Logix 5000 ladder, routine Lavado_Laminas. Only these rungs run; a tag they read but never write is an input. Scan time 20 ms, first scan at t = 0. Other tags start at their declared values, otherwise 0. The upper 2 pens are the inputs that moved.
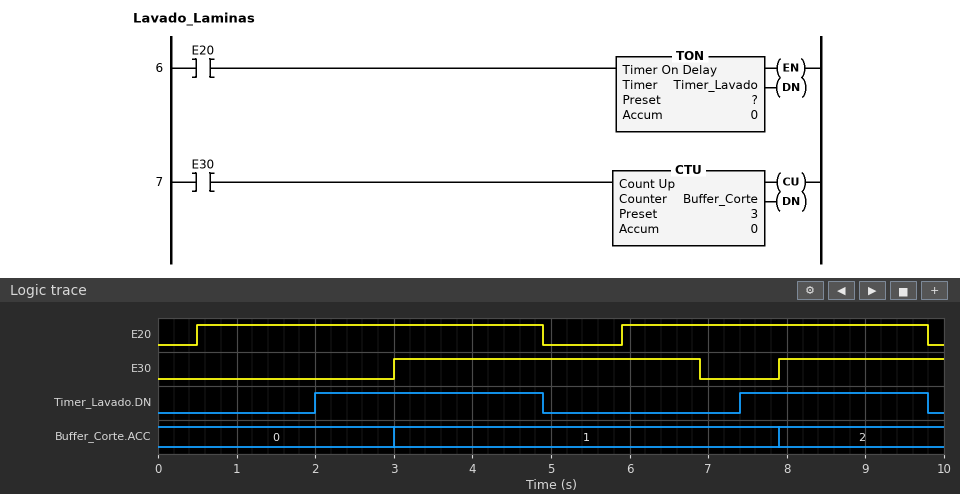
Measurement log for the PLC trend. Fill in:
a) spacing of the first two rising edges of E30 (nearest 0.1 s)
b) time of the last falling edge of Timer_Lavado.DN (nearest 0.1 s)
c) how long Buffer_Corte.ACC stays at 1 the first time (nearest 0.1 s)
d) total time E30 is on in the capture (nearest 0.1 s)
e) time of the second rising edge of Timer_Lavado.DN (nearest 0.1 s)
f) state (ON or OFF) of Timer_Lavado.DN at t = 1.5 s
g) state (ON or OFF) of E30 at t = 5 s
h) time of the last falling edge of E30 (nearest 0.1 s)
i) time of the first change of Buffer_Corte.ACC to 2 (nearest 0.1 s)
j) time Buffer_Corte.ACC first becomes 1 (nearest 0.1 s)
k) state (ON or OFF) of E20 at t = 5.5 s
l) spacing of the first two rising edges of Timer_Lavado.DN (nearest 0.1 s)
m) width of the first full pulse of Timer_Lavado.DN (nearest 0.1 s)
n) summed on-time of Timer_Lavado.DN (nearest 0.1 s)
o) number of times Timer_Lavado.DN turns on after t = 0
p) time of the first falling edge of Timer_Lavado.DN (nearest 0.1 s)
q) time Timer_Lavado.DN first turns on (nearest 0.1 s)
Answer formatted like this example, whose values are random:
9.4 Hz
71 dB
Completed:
4.9 s
9.8 s
4.9 s
6.0 s
7.4 s
OFF
ON
6.9 s
7.9 s
3.0 s
OFF
5.4 s
2.9 s
5.3 s
2
4.9 s
2.0 s
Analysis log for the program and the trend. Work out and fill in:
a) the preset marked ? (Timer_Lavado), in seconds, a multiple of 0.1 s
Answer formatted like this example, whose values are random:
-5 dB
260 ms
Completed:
1.5 s
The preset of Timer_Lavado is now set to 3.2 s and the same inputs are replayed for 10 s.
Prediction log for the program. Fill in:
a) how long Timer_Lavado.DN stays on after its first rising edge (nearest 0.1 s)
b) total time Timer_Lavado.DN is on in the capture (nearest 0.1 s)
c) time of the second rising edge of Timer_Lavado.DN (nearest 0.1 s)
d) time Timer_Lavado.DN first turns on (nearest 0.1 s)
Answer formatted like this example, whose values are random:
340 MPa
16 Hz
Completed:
1.2 s
1.9 s
9.1 s
3.7 s
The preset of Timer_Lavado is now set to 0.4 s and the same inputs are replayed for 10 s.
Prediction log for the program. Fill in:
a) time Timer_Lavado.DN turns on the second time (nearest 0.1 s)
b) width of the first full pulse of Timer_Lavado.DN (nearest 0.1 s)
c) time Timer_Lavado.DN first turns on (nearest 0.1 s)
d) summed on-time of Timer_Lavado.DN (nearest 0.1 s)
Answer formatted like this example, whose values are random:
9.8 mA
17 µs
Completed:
6.3 s
4.0 s
0.9 s
7.5 s
